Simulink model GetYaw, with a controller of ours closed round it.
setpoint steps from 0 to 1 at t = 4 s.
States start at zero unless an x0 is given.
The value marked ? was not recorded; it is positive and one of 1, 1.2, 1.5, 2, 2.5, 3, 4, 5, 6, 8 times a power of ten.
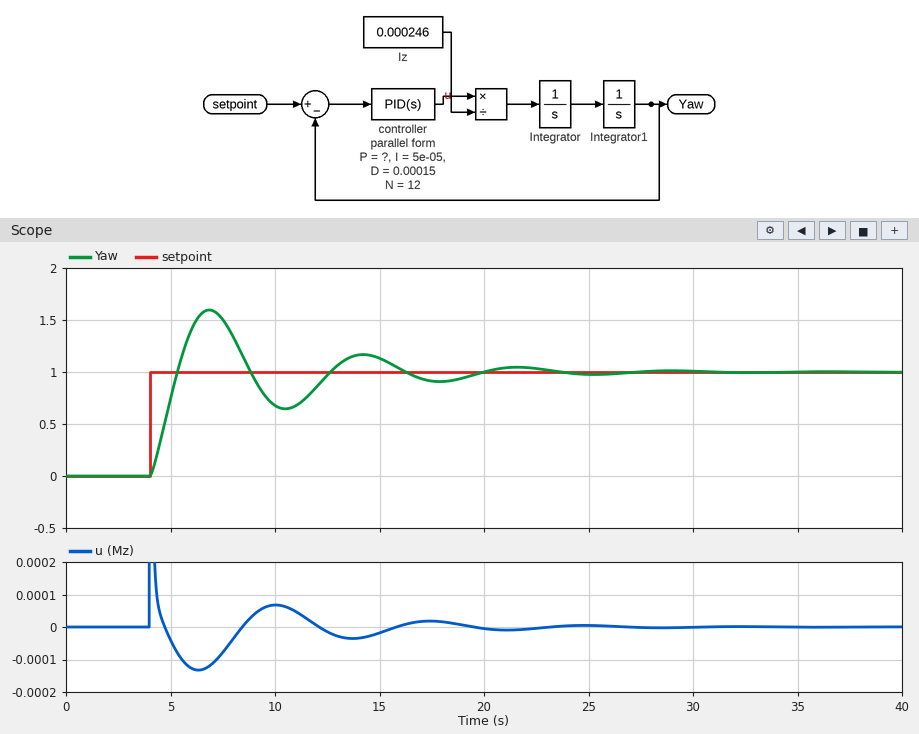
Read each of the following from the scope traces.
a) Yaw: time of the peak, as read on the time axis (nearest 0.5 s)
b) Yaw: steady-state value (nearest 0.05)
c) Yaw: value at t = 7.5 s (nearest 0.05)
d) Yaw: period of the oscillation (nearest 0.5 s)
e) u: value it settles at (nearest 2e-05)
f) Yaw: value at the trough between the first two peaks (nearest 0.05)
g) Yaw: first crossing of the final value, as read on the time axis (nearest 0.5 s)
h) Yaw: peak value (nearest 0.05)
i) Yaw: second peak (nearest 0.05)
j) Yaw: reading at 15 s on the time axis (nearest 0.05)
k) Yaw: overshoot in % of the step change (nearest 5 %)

7.0 s
1.00
1.50
7.5 s
0.00000
0.65
5.5 s
1.60
1.15
1.15
60 %
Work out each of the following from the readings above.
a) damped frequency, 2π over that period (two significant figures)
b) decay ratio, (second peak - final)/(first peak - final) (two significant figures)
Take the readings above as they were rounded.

0.84 rad/s
0.25
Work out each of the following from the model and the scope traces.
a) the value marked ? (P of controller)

0.0002
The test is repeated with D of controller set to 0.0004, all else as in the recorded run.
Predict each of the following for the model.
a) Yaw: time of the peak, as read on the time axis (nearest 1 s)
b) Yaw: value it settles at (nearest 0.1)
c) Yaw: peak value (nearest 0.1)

6 s
1.0
1.2
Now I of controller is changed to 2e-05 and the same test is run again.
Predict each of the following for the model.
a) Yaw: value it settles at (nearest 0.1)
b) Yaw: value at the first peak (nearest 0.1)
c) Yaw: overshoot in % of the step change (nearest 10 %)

1.0
1.5
50 %
